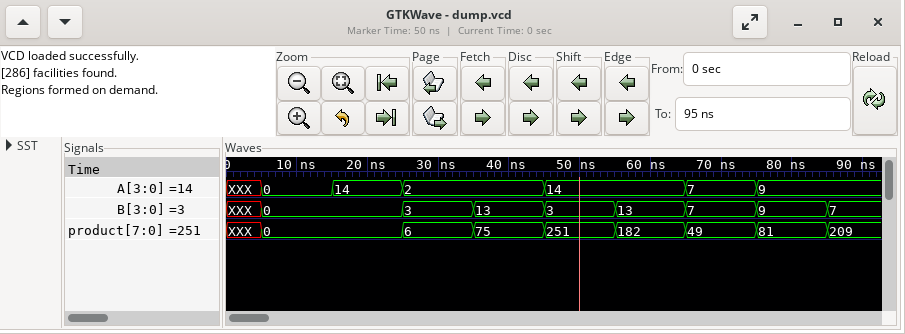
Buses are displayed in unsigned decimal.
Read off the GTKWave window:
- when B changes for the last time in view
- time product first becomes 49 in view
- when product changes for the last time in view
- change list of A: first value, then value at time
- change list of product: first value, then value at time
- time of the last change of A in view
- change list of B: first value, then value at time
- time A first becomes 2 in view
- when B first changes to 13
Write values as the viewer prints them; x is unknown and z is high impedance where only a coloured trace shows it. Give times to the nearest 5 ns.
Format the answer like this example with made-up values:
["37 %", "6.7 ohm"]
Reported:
["85 ns", "65 ns", "85 ns", "XXX, 0 at 5 ns, 14 at 15 ns, 2 at 25 ns, 14 at 45 ns, 7 at 65 ns, 9 at 75 ns", "XXX, 0 at 5 ns, 6 at 25 ns, 75 at 35 ns, 251 at 45 ns, 182 at 55 ns, 49 at 65 ns, 81 at 75 ns, 209 at 85 ns", "75 ns", "XXX, 0 at 5 ns, 3 at 25 ns, 13 at 35 ns, 3 at 45 ns, 13 at 55 ns, 7 at 65 ns, 9 at 75 ns, 7 at 85 ns", "25 ns", "35 ns"]
